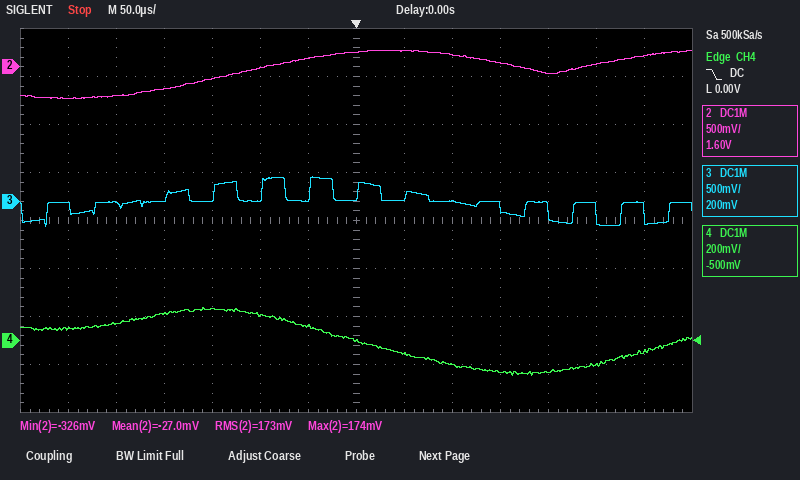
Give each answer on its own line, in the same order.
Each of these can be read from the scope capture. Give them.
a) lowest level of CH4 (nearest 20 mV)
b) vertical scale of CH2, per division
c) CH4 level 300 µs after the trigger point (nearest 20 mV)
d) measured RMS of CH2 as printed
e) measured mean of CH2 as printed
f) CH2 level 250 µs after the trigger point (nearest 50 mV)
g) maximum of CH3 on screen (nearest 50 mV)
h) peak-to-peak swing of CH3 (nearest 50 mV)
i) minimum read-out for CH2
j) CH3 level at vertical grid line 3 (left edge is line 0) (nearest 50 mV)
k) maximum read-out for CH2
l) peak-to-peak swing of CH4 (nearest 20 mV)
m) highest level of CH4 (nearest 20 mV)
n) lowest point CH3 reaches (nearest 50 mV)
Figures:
-140 mV
500 mV
-40 mV
173 mV
-27.0 mV
50 mV
250 mV
500 mV
-326 mV
0 mV
174 mV
280 mV
140 mV
-250 mV
